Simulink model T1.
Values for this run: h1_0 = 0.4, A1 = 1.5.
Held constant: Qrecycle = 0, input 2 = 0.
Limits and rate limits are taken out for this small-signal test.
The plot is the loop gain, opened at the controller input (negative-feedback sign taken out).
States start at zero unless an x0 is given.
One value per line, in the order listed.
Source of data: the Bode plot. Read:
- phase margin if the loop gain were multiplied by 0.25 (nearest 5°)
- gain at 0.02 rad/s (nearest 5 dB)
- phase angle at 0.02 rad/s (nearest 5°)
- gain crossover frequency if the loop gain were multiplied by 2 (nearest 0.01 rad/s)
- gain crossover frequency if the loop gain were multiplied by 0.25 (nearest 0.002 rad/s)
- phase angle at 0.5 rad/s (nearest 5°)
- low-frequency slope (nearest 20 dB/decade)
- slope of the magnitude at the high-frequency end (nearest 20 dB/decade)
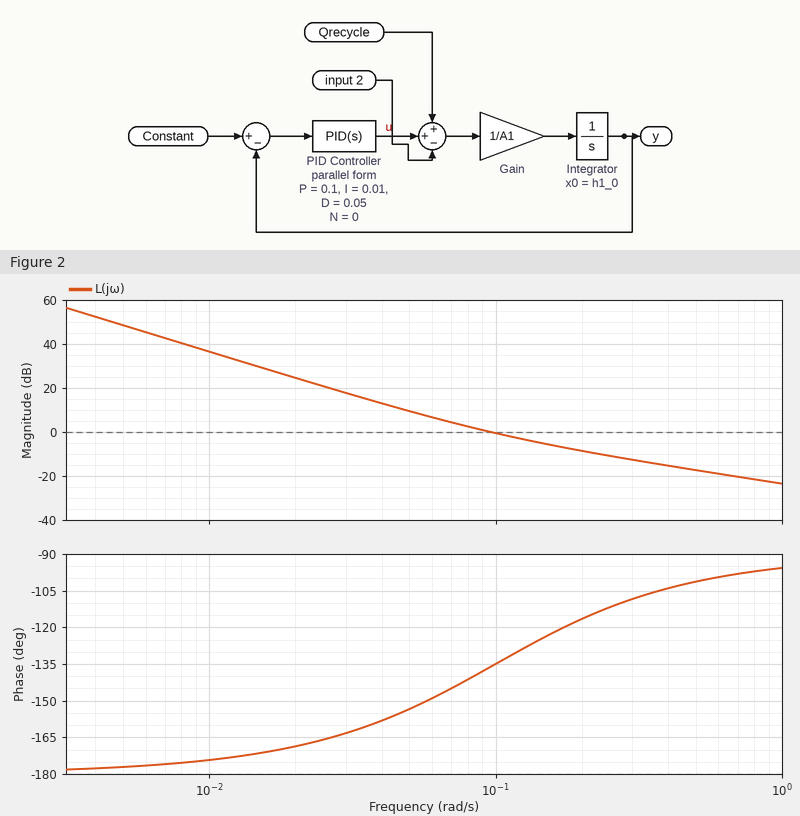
25°
25 dB
-170°
0.16 rad/s
0.042 rad/s
-100°
-40 dB/decade
-20 dB/decade
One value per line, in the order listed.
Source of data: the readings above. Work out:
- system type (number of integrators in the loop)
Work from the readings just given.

2
